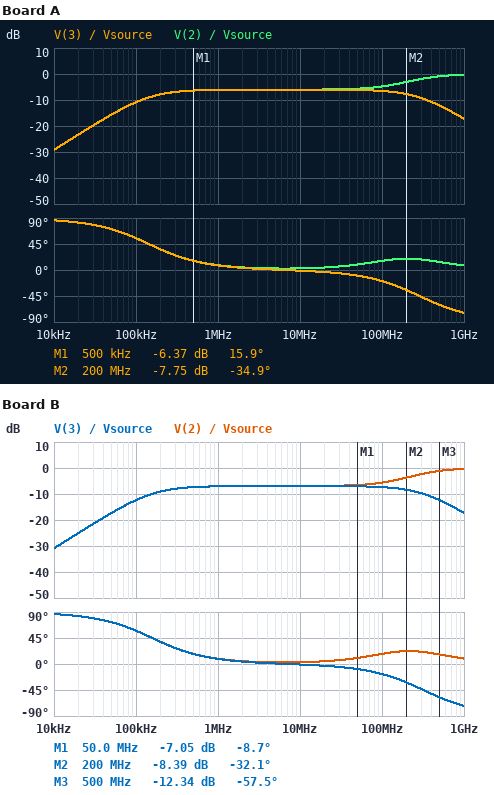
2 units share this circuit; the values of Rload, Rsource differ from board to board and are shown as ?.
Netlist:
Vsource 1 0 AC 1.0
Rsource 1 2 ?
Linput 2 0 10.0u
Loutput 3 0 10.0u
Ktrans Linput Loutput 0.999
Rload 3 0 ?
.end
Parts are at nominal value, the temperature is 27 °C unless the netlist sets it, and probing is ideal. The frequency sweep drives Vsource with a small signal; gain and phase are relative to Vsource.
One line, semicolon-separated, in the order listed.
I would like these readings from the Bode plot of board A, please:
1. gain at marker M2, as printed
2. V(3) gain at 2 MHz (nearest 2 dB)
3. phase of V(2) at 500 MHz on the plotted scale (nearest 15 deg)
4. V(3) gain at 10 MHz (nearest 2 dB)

-7.75 dB; -6 dB; 15 deg; -6 dB
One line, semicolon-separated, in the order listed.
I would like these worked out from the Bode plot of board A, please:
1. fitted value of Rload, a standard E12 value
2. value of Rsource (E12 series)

18 Ω; 18 Ω
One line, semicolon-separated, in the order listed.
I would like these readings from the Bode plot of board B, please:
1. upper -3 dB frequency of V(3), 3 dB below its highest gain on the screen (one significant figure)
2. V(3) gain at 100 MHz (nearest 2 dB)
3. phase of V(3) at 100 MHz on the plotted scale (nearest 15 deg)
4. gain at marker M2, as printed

300 MHz; -8 dB; -15 deg; -8.39 dB
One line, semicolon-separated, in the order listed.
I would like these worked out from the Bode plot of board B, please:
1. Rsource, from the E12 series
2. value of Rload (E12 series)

22 Ω; 18 Ω
